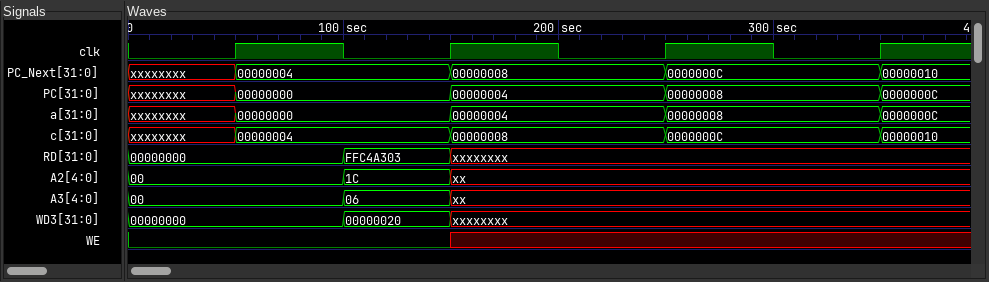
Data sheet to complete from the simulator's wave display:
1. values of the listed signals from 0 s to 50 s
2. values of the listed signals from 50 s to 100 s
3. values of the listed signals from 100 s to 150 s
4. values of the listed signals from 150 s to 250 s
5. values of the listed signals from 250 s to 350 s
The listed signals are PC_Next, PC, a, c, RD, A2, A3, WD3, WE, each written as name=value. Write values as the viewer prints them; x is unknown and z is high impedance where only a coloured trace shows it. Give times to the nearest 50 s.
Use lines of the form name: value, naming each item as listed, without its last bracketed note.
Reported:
values of the listed signals from 0 s to 50 s: PC_Next=xxxxxxxx, PC=xxxxxxxx, a=xxxxxxxx, c=xxxxxxxx, RD=00000000, A2=00, A3=00, WD3=00000000, WE=0
values of the listed signals from 50 s to 100 s: PC_Next=00000004, PC=00000000, a=00000000, c=00000004, RD=00000000, A2=00, A3=00, WD3=00000000, WE=0
values of the listed signals from 100 s to 150 s: PC_Next=00000004, PC=00000000, a=00000000, c=00000004, RD=FFC4A303, A2=1C, A3=06, WD3=00000020, WE=0
values of the listed signals from 150 s to 250 s: PC_Next=00000008, PC=00000004, a=00000004, c=00000008, RD=xxxxxxxx, A2=xx, A3=xx, WD3=xxxxxxxx, WE=x
values of the listed signals from 250 s to 350 s: PC_Next=0000000C, PC=00000008, a=00000008, c=0000000C, RD=xxxxxxxx, A2=xx, A3=xx, WD3=xxxxxxxx, WE=x
